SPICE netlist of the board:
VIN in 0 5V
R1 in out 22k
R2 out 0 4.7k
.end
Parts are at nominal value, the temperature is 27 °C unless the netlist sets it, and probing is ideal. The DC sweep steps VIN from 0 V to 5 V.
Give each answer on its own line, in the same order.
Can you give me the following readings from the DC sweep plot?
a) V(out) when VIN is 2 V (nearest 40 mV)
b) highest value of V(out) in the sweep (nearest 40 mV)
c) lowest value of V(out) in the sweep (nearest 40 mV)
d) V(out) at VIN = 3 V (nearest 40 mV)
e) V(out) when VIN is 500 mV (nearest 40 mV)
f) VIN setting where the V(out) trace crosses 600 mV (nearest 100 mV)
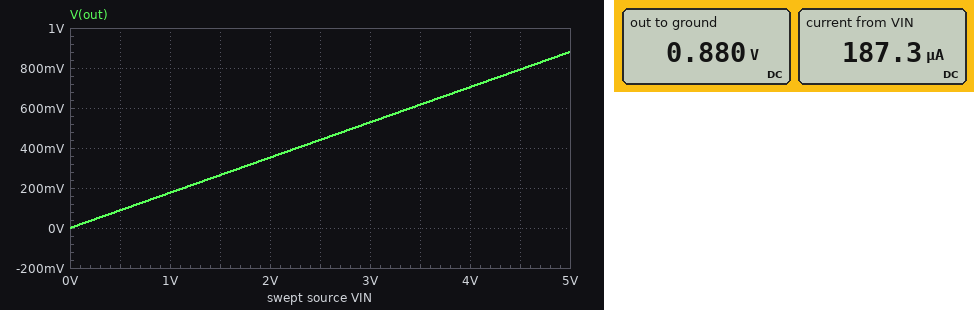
360 mV
880 mV
0 V
520 mV
80 mV
3.4 V
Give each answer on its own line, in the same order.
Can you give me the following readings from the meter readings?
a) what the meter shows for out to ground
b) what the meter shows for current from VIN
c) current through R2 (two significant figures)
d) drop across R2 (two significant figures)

0.880 V
187.3 µA
190 µA
880 mV
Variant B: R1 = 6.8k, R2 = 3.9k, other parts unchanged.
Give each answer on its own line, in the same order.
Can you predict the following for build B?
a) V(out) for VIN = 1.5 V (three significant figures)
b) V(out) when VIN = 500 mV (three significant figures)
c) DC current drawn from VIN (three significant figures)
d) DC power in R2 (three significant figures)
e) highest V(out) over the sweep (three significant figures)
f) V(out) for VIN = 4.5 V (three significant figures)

547 mV
182 mV
467 µA
852 µW
1.82 V
1.64 V
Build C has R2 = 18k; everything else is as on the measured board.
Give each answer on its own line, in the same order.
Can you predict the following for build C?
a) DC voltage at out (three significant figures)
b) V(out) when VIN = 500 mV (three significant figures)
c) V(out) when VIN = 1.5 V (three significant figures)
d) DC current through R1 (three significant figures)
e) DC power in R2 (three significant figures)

2.25 V
225 mV
675 mV
125 µA
281 µW
